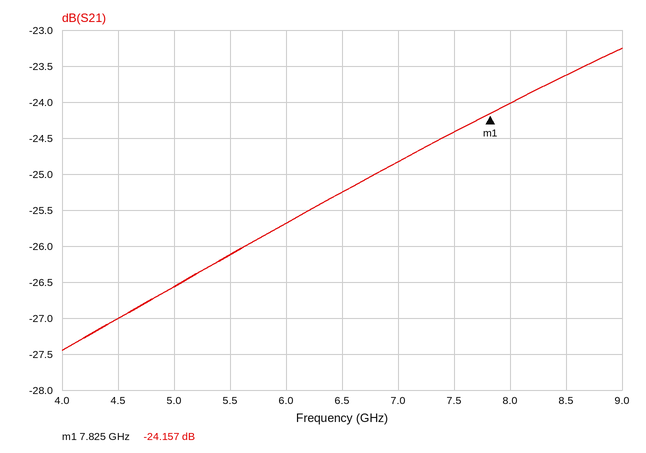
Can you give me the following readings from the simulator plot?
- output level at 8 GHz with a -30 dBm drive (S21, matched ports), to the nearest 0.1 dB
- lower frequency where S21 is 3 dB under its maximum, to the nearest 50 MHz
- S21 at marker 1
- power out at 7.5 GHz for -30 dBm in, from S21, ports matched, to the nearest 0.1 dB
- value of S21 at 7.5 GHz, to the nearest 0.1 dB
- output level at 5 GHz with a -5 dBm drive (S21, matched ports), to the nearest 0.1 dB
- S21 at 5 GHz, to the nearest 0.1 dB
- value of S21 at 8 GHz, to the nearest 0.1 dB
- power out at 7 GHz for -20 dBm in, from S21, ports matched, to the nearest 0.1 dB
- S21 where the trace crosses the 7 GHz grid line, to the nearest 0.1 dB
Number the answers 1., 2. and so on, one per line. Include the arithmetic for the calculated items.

1. -30 dBm + (-24.0 dB) = -54.0 dBm
2. 5.35 GHz
3. -24.157 dB
4. -30 dBm + (-24.4 dB) = -54.4 dBm
5. -24.4 dB
6. -5 dBm + (-26.6 dB) = -31.6 dBm
7. -26.6 dB
8. -24.0 dB
9. -20 dBm + (-24.8 dB) = -44.8 dBm
10. -24.8 dB
